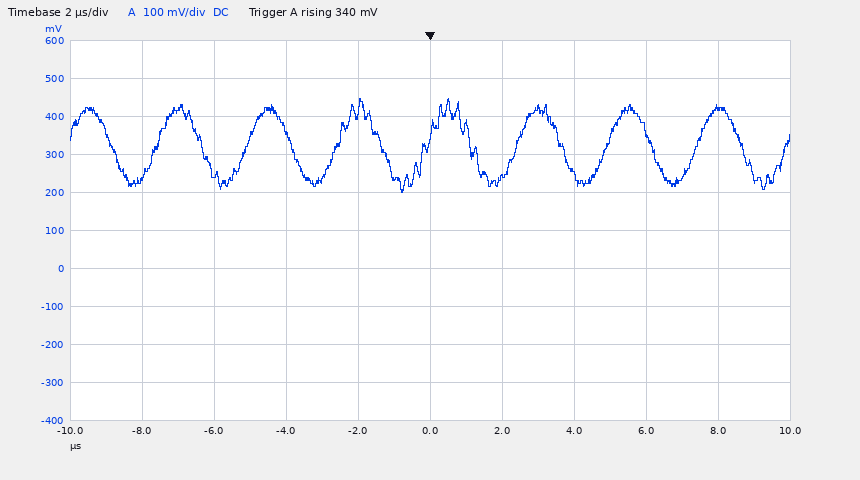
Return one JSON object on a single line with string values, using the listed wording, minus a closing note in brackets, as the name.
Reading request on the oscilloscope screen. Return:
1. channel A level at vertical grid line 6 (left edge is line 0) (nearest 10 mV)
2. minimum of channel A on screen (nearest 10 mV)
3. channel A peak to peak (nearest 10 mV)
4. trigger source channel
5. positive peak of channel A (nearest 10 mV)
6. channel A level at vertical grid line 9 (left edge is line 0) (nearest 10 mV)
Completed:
{"channel A level at vertical grid line 6 (left edge is line 0)": "240 mV", "minimum of channel A on screen": "200 mV", "channel A peak to peak": "250 mV", "trigger source channel": "channel A", "positive peak of channel A": "450 mV", "channel A level at vertical grid line 9 (left edge is line 0)": "420 mV"}
